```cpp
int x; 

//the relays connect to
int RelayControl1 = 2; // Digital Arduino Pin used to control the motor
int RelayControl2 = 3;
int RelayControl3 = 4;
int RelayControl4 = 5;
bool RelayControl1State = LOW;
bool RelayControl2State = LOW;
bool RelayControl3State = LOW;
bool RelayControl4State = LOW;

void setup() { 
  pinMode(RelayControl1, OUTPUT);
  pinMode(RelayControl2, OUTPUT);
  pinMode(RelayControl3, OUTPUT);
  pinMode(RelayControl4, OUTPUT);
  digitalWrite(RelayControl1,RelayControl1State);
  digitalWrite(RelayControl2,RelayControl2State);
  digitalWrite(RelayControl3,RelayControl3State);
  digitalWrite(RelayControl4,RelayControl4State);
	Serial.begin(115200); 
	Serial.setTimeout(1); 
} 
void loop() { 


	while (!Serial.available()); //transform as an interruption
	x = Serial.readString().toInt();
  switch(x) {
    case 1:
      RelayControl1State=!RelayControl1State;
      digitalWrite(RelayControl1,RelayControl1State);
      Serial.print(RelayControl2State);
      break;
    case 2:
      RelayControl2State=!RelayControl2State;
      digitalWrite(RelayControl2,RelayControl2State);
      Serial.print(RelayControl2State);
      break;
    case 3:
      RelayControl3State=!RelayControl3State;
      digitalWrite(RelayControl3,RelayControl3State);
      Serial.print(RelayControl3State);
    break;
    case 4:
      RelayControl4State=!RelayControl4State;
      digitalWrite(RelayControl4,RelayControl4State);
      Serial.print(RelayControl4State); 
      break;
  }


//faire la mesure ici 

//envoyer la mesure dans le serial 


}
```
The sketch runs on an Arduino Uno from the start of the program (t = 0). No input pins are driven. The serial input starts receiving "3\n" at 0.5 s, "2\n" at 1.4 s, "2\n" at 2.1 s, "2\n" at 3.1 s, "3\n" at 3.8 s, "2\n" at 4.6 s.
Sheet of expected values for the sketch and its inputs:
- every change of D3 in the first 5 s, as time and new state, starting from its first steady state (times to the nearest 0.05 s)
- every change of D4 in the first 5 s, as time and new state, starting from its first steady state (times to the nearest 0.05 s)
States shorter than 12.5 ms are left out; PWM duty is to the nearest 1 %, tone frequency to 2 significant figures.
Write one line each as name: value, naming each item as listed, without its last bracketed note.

every change of D3 in the first 5 s, as time and new state, starting from its first steady state: 0 s low; 1.4 s high; 2.1 s low; 3.1 s high; 4.6 s low
every change of D4 in the first 5 s, as time and new state, starting from its first steady state: 0 s low; 0.5 s high; 3.8 s low
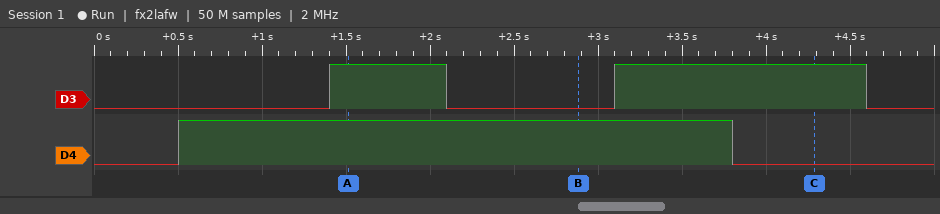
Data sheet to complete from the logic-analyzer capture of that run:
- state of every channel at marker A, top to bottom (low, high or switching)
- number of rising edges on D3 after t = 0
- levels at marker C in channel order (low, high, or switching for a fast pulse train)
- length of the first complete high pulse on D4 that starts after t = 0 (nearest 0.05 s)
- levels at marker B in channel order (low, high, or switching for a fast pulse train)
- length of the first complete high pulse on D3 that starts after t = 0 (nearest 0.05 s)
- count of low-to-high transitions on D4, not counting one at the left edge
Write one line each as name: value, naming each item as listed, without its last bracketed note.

state of every channel at marker A, top to bottom: D3 high, D4 high
number of rising edges on D3 after t = 0: 2
levels at marker C in channel order: D3 high, D4 low
length of the first complete high pulse on D4 that starts after t = 0: 3.30 s
levels at marker B in channel order: D3 low, D4 high
length of the first complete high pulse on D3 that starts after t = 0: 0.70 s
count of low-to-high transitions on D4, not counting one at the left edge: 1
